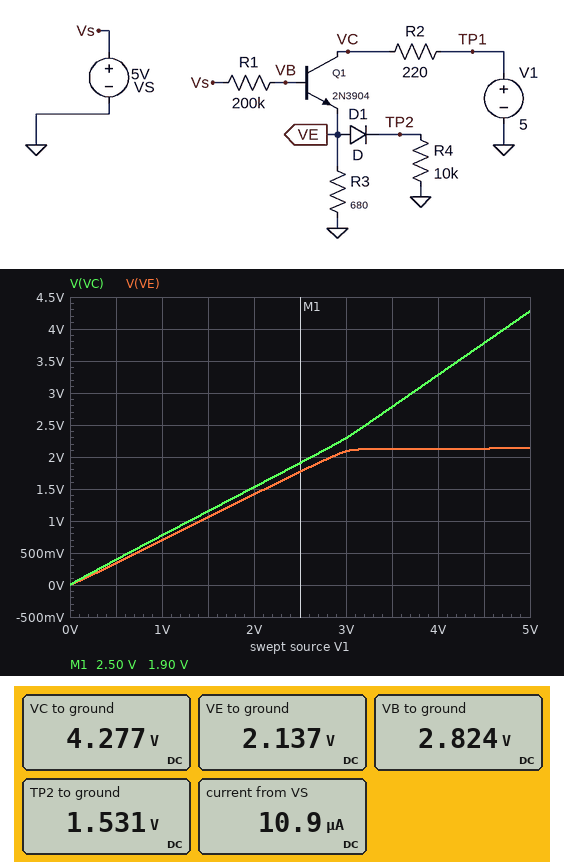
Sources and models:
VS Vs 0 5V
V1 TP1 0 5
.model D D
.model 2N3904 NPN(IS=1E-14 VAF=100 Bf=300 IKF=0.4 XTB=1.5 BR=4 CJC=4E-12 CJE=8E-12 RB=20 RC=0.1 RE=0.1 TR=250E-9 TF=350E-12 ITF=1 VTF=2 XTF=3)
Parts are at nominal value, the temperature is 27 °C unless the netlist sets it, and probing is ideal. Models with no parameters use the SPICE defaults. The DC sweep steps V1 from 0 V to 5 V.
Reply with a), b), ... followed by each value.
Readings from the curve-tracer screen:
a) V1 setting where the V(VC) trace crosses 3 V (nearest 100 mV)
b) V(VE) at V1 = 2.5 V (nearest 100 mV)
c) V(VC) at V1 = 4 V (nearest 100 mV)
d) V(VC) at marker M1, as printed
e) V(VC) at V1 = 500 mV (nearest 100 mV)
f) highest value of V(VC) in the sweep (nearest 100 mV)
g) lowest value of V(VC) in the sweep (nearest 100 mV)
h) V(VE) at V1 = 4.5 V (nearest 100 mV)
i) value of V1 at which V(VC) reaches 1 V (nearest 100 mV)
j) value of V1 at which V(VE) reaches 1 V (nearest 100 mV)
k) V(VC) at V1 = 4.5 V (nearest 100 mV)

a) 3.7 V
b) 1.8 V
c) 3.3 V
d) 1.90 V
e) 400 mV
f) 4.3 V
g) 0 V
h) 2.1 V
i) 1.3 V
j) 1.4 V
k) 3.8 V
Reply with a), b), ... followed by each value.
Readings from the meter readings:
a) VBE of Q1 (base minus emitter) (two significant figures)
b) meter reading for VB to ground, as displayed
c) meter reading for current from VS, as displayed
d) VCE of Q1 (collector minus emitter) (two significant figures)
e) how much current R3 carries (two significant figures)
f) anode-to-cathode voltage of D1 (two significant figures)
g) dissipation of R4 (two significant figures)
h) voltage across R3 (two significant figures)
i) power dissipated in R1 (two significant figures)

a) 690 mV
b) 2.824 V
c) 10.9 µA
d) 2.1 V
e) 3.1 mA
f) 610 mV
g) 230 µW
h) 2.1 V
i) 24 µW
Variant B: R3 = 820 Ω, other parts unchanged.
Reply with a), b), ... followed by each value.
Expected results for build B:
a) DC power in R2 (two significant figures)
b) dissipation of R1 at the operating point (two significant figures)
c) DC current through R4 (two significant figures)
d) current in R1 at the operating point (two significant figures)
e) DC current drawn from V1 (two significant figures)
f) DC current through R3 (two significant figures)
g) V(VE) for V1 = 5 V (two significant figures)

a) 2.0 mW
b) 20 µW
c) 170 µA
d) 9.9 µA
e) 3.0 mA
f) 2.8 mA
g) 2.3 V
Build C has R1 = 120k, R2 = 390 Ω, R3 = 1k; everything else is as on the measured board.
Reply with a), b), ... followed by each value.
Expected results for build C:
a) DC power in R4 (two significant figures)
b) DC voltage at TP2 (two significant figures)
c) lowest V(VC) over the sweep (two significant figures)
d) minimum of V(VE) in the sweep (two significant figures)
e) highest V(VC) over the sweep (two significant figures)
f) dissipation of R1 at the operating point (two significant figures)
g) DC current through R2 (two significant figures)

a) 570 µW
b) 2.4 V
c) 11 mV
d) 9.2 mV
e) 3.7 V
f) 14 µW
g) 3.2 mA
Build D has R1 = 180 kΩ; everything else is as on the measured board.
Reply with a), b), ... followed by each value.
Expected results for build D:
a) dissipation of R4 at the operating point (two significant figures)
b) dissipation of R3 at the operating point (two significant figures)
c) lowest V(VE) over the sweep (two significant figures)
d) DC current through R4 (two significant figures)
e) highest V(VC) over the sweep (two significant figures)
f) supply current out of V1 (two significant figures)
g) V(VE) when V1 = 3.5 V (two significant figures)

a) 270 µW
b) 7.4 mW
c) 3.2 mV
d) 160 µA
e) 4.2 V
f) 3.5 mA
g) 2.2 V
